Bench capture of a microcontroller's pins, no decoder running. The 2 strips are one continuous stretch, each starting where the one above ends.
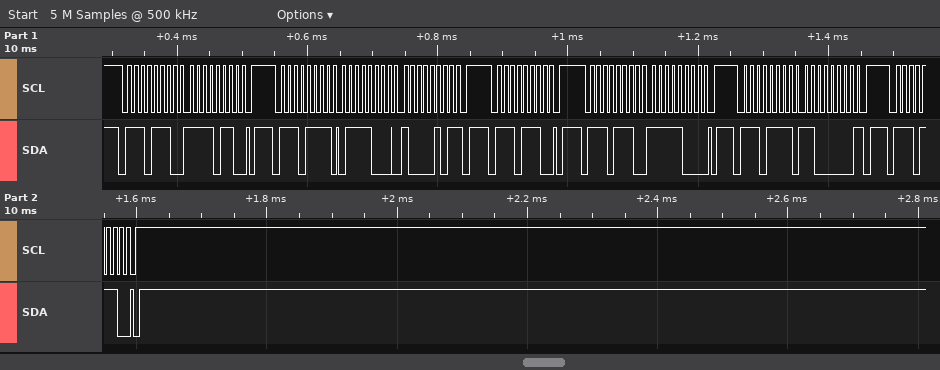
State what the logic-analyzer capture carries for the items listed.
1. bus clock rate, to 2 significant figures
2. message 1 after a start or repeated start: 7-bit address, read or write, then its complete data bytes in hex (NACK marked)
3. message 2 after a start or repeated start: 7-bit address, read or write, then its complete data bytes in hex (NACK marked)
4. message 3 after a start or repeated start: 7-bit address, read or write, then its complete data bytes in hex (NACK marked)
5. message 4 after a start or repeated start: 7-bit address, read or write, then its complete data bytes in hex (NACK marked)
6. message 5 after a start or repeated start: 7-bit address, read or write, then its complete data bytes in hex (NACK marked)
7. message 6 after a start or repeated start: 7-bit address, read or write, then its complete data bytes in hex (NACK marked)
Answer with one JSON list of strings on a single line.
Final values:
["100 kHz", "0x77 write: F6", "0x77 read: 78 85 NACK", "0x77 write", "0x77 write: F8", "0x77 read: C0 NACK", "0x77 write"]
